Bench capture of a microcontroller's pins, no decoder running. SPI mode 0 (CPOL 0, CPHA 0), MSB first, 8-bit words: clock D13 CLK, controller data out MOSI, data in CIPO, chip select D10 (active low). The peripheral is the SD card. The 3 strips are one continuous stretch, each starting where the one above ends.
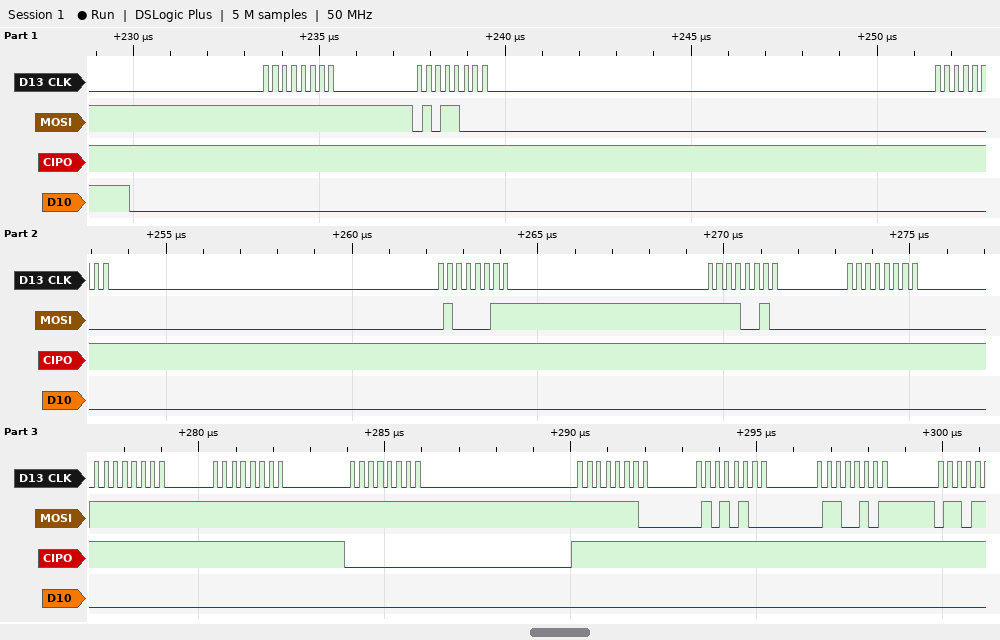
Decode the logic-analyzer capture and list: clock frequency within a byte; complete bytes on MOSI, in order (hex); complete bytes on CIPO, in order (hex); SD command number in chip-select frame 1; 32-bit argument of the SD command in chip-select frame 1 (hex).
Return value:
4 MHz
FF 58 00 43 F2 00 FF FF FF FE 54 65
FF FF FF FF FF FF FF FF 00 FF FF FF
CMD24
0x0043F200
